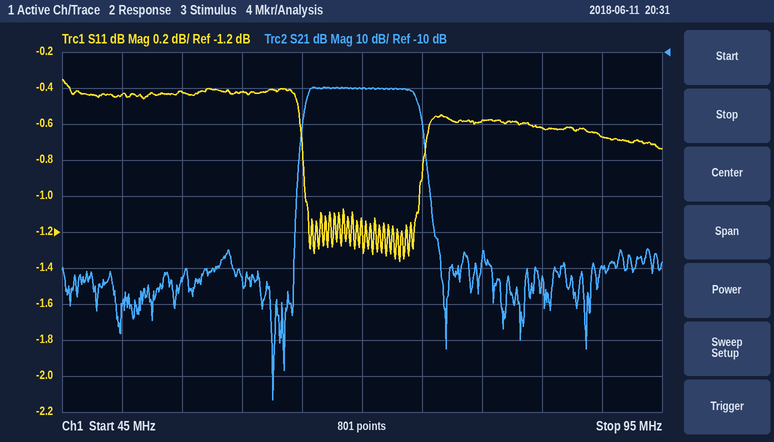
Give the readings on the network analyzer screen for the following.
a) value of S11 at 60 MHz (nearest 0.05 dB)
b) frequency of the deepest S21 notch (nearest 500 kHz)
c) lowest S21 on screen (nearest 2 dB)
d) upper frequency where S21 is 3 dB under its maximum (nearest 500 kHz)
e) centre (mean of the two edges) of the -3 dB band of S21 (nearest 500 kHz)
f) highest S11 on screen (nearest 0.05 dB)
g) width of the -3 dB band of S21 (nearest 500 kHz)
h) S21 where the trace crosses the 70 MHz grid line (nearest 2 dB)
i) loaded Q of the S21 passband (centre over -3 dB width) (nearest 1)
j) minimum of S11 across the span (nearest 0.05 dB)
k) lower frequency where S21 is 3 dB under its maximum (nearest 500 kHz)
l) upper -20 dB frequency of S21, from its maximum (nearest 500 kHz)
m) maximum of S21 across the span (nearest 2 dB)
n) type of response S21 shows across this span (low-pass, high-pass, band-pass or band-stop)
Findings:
-0.40 dB
62.5 MHz
-106 dB
74.5 MHz
70.0 MHz
-0.35 dB
9.0 MHz
-20 dB
8
-1.35 dB
65.5 MHz
75.5 MHz
-20 dB
band-pass
